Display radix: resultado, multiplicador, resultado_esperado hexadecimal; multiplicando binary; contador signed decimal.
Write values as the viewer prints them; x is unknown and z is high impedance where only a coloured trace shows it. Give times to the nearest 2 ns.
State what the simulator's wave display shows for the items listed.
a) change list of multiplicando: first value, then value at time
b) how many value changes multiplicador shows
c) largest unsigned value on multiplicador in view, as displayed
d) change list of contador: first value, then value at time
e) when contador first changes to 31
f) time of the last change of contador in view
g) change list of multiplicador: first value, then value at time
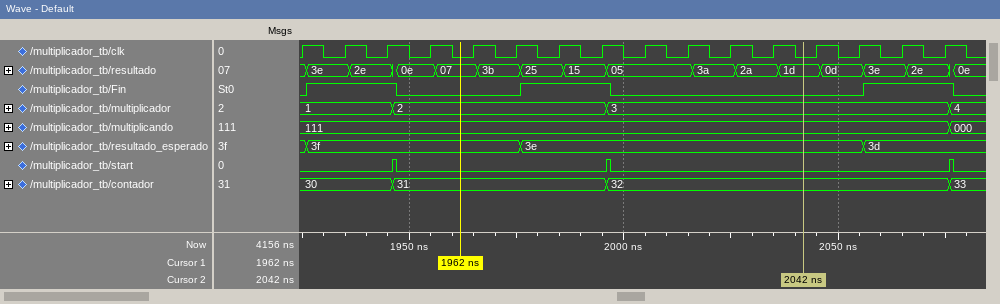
111, 000 at 2076 ns
3
4
30, 31 at 1946 ns, 32 at 1996 ns, 33 at 2076 ns
1946 ns
2076 ns
1, 2 at 1946 ns, 3 at 1996 ns, 4 at 2076 ns
